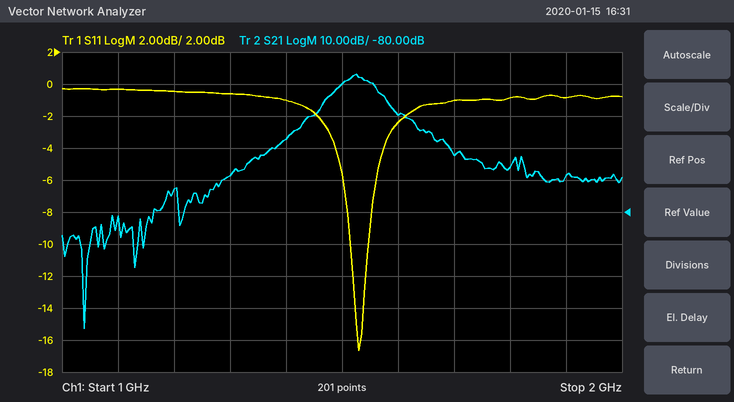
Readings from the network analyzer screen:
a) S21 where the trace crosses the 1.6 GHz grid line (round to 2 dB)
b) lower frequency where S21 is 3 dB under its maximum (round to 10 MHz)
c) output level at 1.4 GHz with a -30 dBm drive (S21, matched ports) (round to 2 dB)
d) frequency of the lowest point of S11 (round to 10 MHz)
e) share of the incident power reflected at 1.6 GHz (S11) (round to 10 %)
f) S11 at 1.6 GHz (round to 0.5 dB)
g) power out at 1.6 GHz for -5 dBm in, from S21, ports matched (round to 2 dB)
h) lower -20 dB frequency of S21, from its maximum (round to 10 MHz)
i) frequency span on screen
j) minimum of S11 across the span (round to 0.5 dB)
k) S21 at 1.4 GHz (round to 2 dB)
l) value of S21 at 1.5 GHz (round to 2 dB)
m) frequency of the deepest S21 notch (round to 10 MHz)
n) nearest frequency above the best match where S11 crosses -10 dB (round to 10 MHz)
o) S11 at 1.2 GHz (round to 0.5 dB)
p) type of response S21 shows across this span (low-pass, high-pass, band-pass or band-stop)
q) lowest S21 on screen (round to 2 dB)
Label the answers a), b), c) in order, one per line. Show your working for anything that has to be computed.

a) -50 dB
b) 1.50 GHz
c) -30 dBm + (-58 dB) = -88 dBm
d) 1.53 GHz
e) 10^(-2.5/10) ≈ 56.2 %, so 60 % to the nearest 10 %
f) -2.5 dB
g) -5 dBm + (-50 dB) = -54 dBm
h) 1.40 GHz
i) 1 GHz
j) -16.5 dB
k) -58 dB
l) -40 dB
m) 1.04 GHz
n) 1.55 GHz
o) -0.5 dB
p) band-pass
q) -116 dB
